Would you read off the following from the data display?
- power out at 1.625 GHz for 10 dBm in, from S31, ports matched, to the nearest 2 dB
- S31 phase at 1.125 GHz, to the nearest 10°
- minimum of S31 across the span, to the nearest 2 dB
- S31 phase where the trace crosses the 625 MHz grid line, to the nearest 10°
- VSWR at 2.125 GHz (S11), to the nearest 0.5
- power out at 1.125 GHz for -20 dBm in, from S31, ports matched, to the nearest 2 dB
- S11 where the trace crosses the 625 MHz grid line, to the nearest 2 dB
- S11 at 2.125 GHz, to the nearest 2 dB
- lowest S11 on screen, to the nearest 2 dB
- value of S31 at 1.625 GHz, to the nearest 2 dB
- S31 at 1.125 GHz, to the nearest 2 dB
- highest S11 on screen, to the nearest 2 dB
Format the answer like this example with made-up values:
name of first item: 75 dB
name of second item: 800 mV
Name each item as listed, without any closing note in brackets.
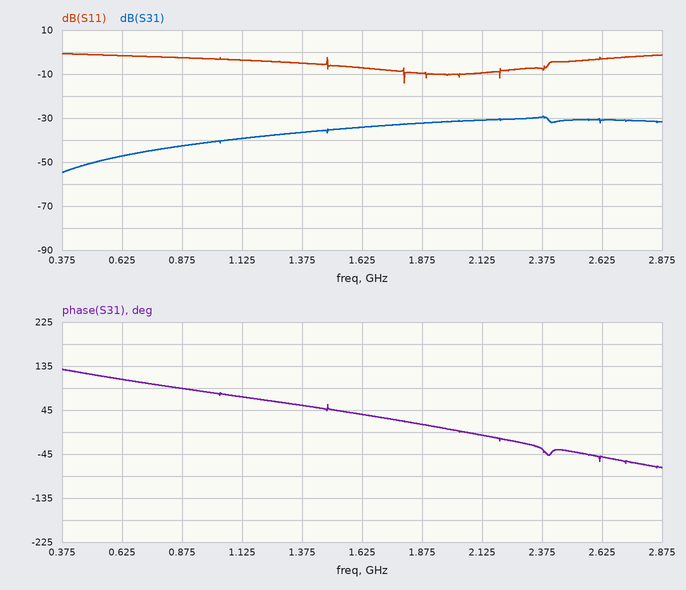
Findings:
power out at 1.625 GHz for 10 dBm in, from S31, ports matched, to the nearest 2 dB: -24 dBm
S31 phase at 1.125 GHz, to the nearest 10°: 70°
minimum of S31 across the span, to the nearest 2 dB: -54 dB
S31 phase where the trace crosses the 625 MHz grid line, to the nearest 10°: 110°
VSWR at 2.125 GHz (S11), to the nearest 0.5: 2.0
power out at 1.125 GHz for -20 dBm in, from S31, ports matched, to the nearest 2 dB: -60 dBm
S11 where the trace crosses the 625 MHz grid line, to the nearest 2 dB: -2 dB
S11 at 2.125 GHz, to the nearest 2 dB: -10 dB
lowest S11 on screen, to the nearest 2 dB: -14 dB
value of S31 at 1.625 GHz, to the nearest 2 dB: -34 dB
S31 at 1.125 GHz, to the nearest 2 dB: -40 dB
highest S11 on screen, to the nearest 2 dB: 0 dB
